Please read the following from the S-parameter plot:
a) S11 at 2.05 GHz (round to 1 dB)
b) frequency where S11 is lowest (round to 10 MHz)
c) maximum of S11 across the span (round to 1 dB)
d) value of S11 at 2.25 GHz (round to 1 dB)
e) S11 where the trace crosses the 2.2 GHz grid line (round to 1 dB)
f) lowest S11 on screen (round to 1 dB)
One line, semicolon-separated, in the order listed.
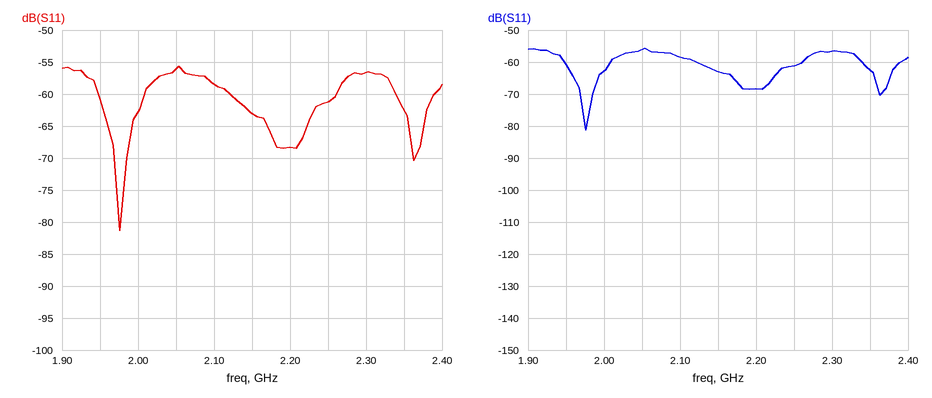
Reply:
-56 dB; 1.98 GHz; -56 dB; -61 dB; -68 dB; -81 dB
